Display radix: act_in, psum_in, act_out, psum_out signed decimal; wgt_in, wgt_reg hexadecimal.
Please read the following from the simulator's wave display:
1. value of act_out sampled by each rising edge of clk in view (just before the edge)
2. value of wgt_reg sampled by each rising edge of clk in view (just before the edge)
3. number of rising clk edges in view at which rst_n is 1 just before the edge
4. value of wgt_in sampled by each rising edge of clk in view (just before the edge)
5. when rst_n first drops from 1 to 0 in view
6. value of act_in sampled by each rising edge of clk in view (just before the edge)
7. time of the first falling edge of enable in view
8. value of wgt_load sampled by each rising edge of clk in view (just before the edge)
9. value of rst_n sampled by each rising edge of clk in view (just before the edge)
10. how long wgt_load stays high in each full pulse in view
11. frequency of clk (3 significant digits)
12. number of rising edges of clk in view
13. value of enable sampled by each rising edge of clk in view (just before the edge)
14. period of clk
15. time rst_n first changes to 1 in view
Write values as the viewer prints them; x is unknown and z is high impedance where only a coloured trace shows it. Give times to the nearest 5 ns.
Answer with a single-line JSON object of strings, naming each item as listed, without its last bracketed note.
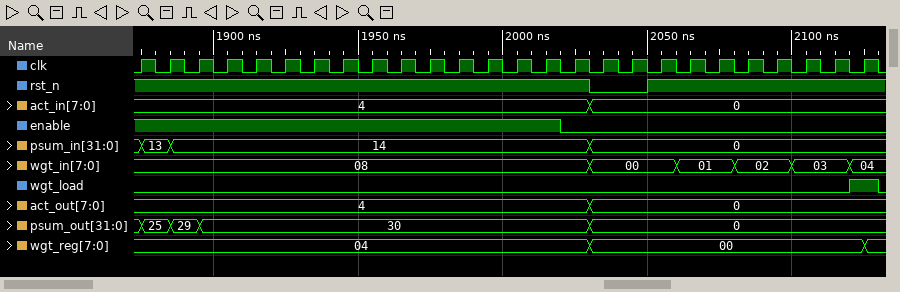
{"value of act_out sampled by each rising edge of clk in view": "4, 4, 4, 4, 4, 4, 4, 4, 4, 4, 4, 4, 4, 4, 4, 4, 0, 0, 0, 0, 0, 0, 0, 0, 0, 0", "value of wgt_reg sampled by each rising edge of clk in view": "04, 04, 04, 04, 04, 04, 04, 04, 04, 04, 04, 04, 04, 04, 04, 04, 00, 00, 00, 00, 00, 00, 00, 00, 00, 00", "number of rising clk edges in view at which rst_n is 1 just before the edge": "24", "value of wgt_in sampled by each rising edge of clk in view": "08, 08, 08, 08, 08, 08, 08, 08, 08, 08, 08, 08, 08, 08, 08, 08, 00, 00, 00, 01, 01, 02, 02, 03, 03, 04", "when rst_n first drops from 1 to 0 in view": "2030 ns", "value of act_in sampled by each rising edge of clk in view": "4, 4, 4, 4, 4, 4, 4, 4, 4, 4, 4, 4, 4, 4, 4, 4, 0, 0, 0, 0, 0, 0, 0, 0, 0, 0", "time of the first falling edge of enable in view": "2020 ns", "value of wgt_load sampled by each rising edge of clk in view": "0 0 0 0 0 0 0 0 0 0 0 0 0 0 0 0 0 0 0 0 0 0 0 0 0 1", "value of rst_n sampled by each rising edge of clk in view": "1 1 1 1 1 1 1 1 1 1 1 1 1 1 1 1 0 0 1 1 1 1 1 1 1 1", "how long wgt_load stays high in each full pulse in view": "10 ns", "frequency of clk": "100 MHz", "number of rising edges of clk in view": "26", "value of enable sampled by each rising edge of clk in view": "1 1 1 1 1 1 1 1 1 1 1 1 1 1 1 0 0 0 0 0 0 0 0 0 0 0", "period of clk": "10 ns", "time rst_n first changes to 1 in view": "2050 ns"}
